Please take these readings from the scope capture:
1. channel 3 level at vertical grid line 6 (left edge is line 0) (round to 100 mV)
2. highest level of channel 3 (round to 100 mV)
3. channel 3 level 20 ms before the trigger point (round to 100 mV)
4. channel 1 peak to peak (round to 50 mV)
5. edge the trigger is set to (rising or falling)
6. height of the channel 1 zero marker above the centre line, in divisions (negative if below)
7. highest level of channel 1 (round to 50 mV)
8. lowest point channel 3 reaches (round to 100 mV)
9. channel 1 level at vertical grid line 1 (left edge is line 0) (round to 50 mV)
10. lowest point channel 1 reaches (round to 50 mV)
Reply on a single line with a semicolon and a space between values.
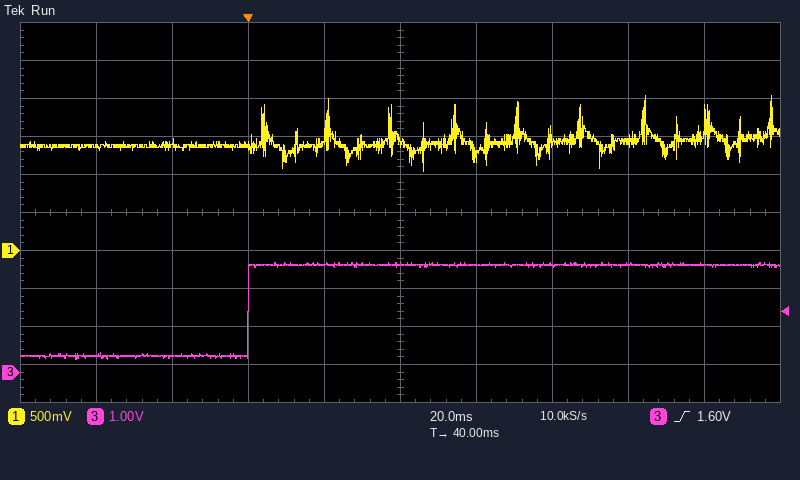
2.8 V; 2.9 V; 400 mV; 1.00 V; rising; -1.0 div; 2.05 V; 300 mV; 1.35 V; 1.05 V
